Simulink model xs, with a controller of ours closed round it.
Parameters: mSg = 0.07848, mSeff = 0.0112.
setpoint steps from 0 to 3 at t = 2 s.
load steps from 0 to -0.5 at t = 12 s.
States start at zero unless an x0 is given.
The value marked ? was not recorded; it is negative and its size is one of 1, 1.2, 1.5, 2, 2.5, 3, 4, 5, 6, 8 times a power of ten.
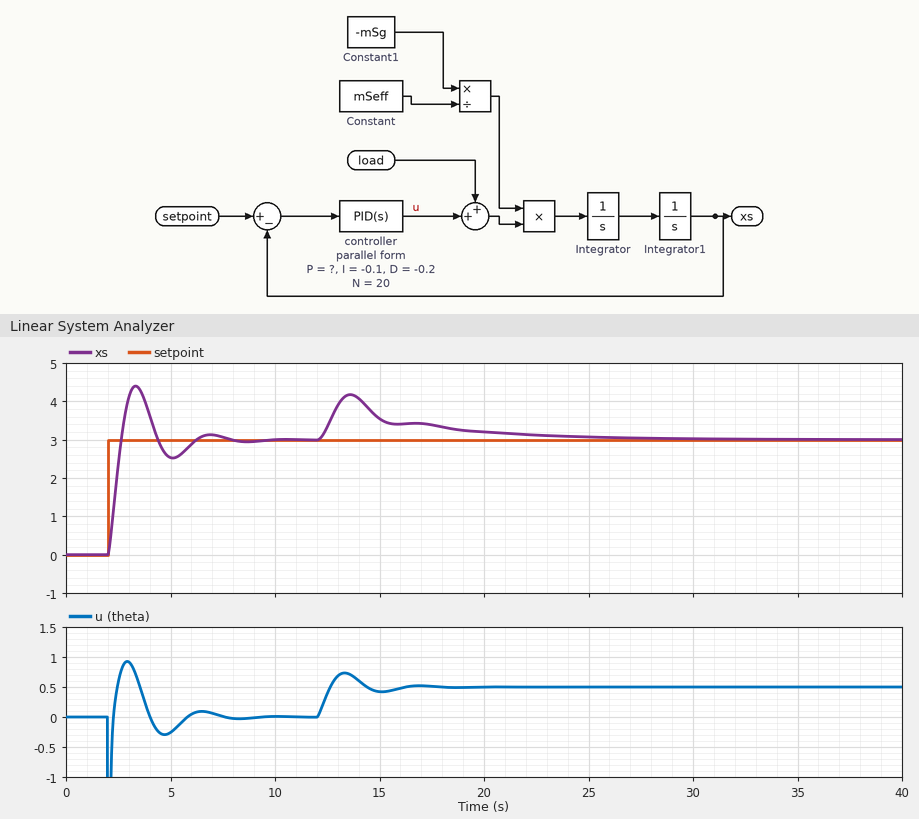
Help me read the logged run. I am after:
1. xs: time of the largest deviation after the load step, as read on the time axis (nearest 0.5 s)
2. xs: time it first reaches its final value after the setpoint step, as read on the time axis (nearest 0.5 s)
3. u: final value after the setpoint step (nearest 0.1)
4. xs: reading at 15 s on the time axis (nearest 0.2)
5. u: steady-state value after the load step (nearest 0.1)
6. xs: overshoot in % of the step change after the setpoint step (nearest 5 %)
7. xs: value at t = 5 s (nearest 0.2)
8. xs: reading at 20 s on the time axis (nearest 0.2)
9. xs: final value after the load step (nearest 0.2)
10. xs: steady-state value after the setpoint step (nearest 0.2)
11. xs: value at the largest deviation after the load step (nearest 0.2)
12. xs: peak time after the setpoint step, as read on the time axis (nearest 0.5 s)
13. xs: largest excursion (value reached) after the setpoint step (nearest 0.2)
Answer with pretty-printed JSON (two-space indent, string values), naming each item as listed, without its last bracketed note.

{
  "xs: time of the largest deviation after the load step, as read on the time axis": "13.5 s",
  "xs: time it first reaches its final value after the setpoint step, as read on the time axis": "2.5 s",
  "u: final value after the setpoint step": "0.0",
  "xs: reading at 15 s on the time axis": "3.6",
  "u: steady-state value after the load step": "0.5",
  "xs: overshoot in % of the step change after the setpoint step": "45 %",
  "xs: value at t = 5 s": "2.6",
  "xs: reading at 20 s on the time axis": "3.2",
  "xs: final value after the load step": "3.0",
  "xs: steady-state value after the setpoint step": "3.0",
  "xs: value at the largest deviation after the load step": "4.2",
  "xs: peak time after the setpoint step, as read on the time axis": "3.5 s",
  "xs: largest excursion (value reached) after the setpoint step": "4.4"
}
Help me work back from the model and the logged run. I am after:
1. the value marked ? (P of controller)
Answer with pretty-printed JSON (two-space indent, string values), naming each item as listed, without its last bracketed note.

{
  "the value marked ?": "-0.5"
}
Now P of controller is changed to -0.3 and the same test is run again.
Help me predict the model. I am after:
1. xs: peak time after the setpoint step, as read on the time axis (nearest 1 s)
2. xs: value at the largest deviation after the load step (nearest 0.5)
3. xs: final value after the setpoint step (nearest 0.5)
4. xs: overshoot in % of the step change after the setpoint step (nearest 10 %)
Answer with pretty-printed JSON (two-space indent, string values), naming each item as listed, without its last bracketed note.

{
  "xs: peak time after the setpoint step, as read on the time axis": "4 s",
  "xs: value at the largest deviation after the load step": "4.5",
  "xs: final value after the setpoint step": "3.0",
  "xs: overshoot in % of the step change after the setpoint step": "40 %"
}
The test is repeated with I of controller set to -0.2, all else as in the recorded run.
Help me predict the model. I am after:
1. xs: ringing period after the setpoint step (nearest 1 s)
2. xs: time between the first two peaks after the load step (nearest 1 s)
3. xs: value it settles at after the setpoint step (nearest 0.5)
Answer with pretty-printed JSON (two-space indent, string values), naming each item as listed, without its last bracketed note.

{
  "xs: ringing period after the setpoint step": "4 s",
  "xs: time between the first two peaks after the load step": "4 s",
  "xs: value it settles at after the setpoint step": "3.0"
}
